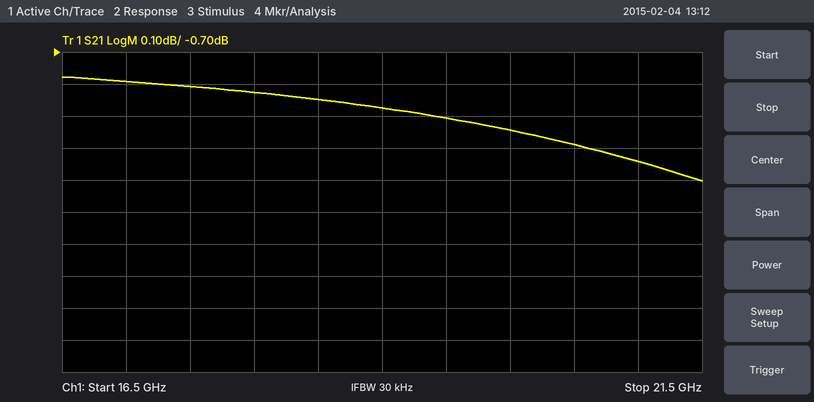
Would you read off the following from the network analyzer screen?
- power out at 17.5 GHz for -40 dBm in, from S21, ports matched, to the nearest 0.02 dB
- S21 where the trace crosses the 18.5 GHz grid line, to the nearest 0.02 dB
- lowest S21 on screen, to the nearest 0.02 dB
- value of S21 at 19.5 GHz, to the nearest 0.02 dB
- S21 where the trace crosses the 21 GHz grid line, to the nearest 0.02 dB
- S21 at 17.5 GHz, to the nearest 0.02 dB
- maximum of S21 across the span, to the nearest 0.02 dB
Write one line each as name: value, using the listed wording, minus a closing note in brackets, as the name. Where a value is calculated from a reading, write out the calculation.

power out at 17.5 GHz for -40 dBm in, from S21, ports matched, to the nearest 0.02 dB: -40 dBm + (-0.80 dB) = -40.80 dBm
S21 where the trace crosses the 18.5 GHz grid line, to the nearest 0.02 dB: -0.84 dB
lowest S21 on screen, to the nearest 0.02 dB: -1.10 dB
value of S21 at 19.5 GHz, to the nearest 0.02 dB: -0.90 dB
S21 where the trace crosses the 21 GHz grid line, to the nearest 0.02 dB: -1.04 dB
S21 at 17.5 GHz, to the nearest 0.02 dB: -0.80 dB
maximum of S21 across the span, to the nearest 0.02 dB: -0.78 dB
